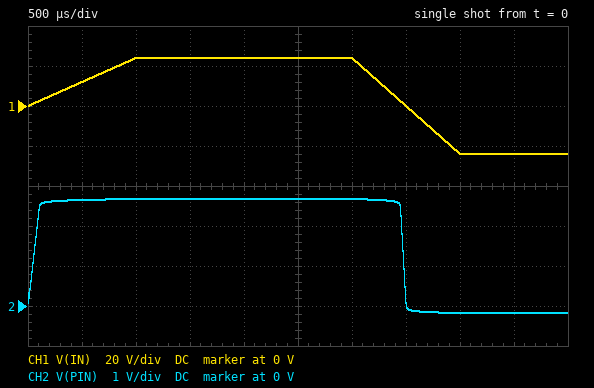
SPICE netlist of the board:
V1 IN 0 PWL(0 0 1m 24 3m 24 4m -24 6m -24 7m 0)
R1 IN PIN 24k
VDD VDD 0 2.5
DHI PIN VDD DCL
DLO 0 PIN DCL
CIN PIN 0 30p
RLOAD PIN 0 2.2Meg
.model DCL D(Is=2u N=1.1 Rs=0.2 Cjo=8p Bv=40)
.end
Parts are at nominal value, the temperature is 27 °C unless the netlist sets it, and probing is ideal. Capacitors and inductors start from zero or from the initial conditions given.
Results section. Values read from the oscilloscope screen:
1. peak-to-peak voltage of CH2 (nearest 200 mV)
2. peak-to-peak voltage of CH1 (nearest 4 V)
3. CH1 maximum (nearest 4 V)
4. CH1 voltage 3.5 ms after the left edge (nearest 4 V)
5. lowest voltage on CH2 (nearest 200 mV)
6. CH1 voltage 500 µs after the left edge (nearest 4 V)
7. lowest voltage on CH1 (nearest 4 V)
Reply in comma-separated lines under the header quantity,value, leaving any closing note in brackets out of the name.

quantity,value
peak-to-peak voltage of CH2,2.8 V
peak-to-peak voltage of CH1,48 V
CH1 maximum,24 V
CH1 voltage 3.5 ms after the left edge,0 V
lowest voltage on CH2,-200 mV
CH1 voltage 500 µs after the left edge,12 V
lowest voltage on CH1,-24 V
